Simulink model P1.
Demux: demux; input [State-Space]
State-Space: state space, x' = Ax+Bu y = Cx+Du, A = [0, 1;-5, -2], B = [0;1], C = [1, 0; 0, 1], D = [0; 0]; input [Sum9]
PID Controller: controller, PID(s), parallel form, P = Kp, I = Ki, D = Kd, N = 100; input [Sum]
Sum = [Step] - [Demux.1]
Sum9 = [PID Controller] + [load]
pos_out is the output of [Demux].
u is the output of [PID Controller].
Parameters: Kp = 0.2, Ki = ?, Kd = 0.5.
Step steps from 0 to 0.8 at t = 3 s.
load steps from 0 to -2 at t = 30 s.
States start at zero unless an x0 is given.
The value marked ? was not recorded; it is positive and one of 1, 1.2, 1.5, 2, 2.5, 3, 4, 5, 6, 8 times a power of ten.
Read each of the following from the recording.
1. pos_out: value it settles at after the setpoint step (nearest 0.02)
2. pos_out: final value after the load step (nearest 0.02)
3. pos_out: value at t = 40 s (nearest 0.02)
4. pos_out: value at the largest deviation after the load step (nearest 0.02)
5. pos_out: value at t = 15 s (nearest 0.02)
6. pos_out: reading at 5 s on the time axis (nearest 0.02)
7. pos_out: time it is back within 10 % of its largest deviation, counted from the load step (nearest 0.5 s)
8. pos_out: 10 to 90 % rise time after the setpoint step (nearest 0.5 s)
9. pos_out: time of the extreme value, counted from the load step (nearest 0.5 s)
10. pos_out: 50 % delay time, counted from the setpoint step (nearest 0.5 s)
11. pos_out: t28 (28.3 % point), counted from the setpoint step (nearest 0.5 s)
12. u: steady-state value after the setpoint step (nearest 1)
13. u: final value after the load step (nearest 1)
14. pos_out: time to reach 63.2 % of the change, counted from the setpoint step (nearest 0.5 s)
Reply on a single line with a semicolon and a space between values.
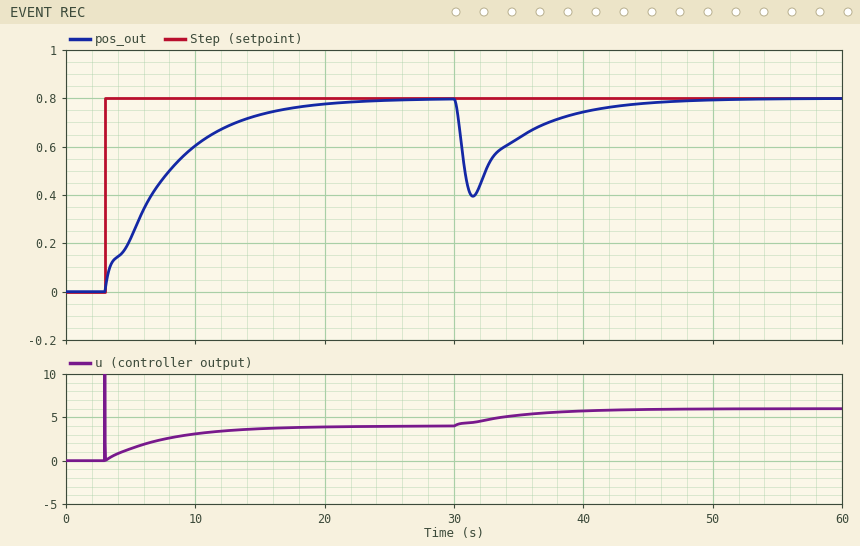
0.80; 0.80; 0.74; 0.40; 0.74; 0.22; 11.5 s; 11.0 s; 1.5 s; 3.5 s; 2.0 s; 4; 6; 5.0 s
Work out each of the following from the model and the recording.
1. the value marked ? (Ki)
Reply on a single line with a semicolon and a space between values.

1
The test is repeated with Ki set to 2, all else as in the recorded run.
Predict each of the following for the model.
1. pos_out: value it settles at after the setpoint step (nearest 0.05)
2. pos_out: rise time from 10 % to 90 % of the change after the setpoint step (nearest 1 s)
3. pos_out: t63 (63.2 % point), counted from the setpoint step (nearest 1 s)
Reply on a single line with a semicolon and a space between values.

0.80; 5 s; 3 s
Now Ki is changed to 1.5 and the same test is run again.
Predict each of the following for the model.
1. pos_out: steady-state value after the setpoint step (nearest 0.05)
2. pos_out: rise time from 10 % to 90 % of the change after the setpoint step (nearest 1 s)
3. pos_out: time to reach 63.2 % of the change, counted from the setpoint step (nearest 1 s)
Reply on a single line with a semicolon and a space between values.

0.80; 7 s; 3 s
